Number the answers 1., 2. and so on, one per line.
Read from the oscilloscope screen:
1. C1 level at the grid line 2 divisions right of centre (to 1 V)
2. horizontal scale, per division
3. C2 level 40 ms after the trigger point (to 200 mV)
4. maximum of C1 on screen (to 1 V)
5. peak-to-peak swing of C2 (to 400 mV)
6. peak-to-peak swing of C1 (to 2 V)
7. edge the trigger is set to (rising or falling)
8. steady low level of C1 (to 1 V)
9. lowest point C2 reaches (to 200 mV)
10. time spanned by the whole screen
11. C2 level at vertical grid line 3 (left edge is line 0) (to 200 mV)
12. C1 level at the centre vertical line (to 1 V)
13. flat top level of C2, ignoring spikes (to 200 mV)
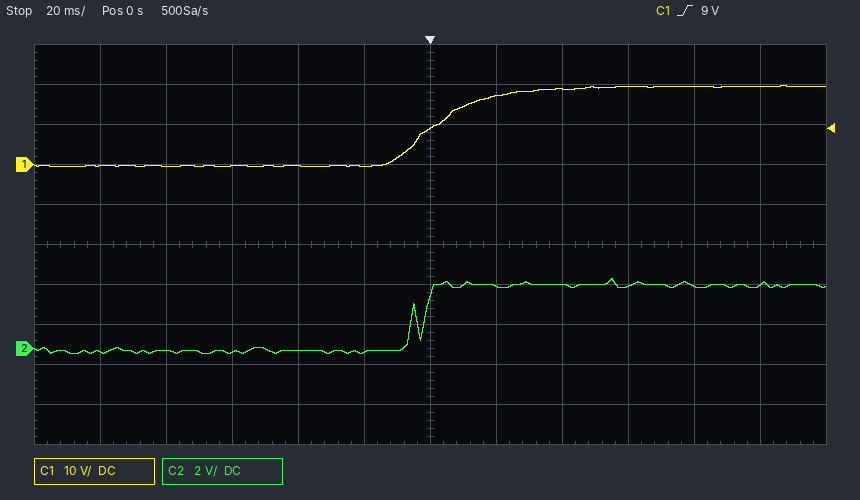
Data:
1. 19 V
2. 20 ms
3. 3.2 V
4. 20 V
5. 3.6 V
6. 20 V
7. rising
8. 0 V
9. -200 mV
10. 240 ms
11. -200 mV
12. 9 V
13. 3.2 V
